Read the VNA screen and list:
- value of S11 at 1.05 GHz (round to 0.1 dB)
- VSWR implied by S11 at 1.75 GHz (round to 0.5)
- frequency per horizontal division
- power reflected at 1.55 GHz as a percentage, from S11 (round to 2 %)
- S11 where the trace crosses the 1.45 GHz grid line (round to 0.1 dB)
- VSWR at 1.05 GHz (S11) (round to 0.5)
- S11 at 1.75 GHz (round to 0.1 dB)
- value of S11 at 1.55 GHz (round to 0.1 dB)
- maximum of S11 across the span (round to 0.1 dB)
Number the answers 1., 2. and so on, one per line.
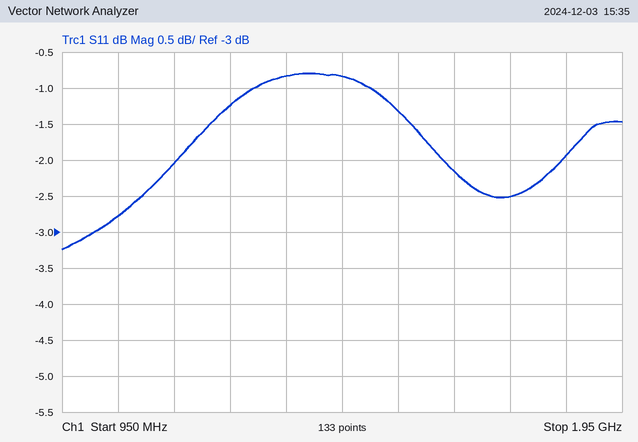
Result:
1. -2.8 dB
2. 7.0
3. 100 MHz
4. 74 %
5. -0.8 dB
6. 6.5
7. -2.5 dB
8. -1.3 dB
9. -0.8 dB
